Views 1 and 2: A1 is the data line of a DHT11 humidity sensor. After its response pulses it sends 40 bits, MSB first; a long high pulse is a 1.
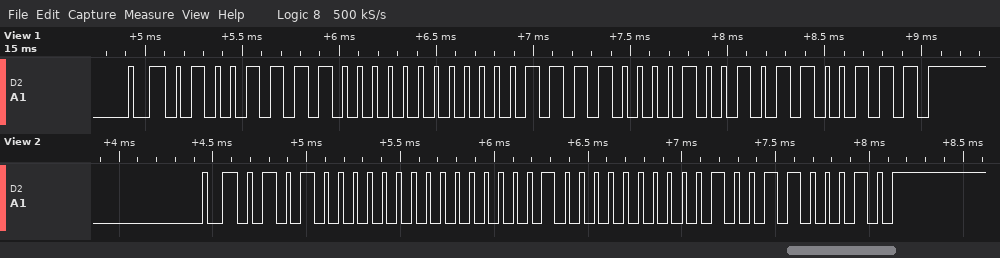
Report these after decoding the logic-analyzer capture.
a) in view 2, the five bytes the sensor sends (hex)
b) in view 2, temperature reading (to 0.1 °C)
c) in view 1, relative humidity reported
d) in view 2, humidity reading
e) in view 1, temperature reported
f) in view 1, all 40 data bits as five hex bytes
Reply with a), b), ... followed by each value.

a) 50 00 10 02 62
b) 16.2 °C
c) 79 %
d) 80 %
e) 15.9 °C
f) 4F 00 0F 09 67
